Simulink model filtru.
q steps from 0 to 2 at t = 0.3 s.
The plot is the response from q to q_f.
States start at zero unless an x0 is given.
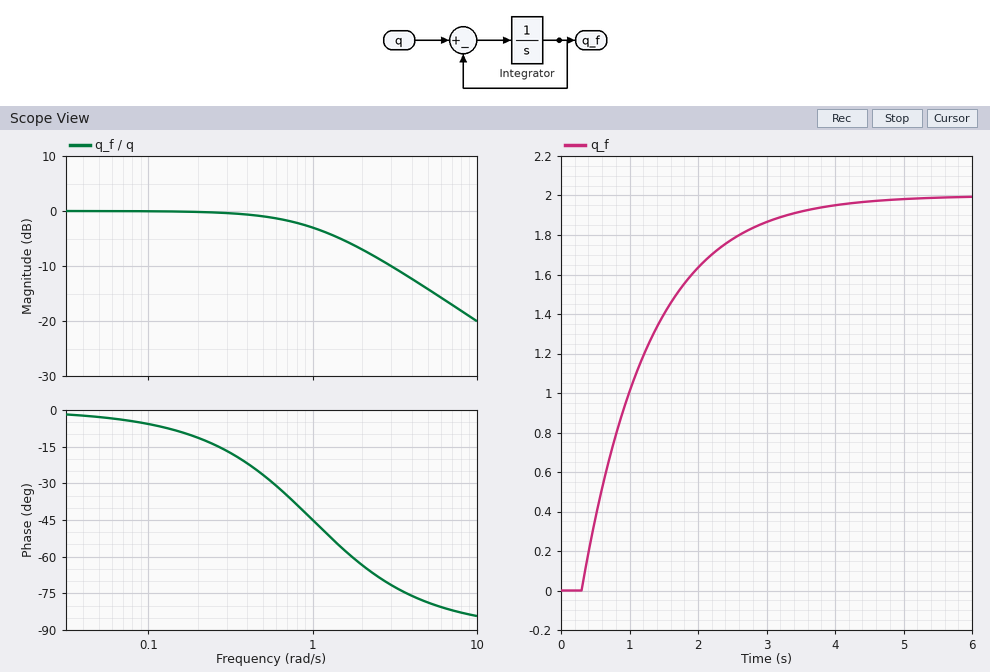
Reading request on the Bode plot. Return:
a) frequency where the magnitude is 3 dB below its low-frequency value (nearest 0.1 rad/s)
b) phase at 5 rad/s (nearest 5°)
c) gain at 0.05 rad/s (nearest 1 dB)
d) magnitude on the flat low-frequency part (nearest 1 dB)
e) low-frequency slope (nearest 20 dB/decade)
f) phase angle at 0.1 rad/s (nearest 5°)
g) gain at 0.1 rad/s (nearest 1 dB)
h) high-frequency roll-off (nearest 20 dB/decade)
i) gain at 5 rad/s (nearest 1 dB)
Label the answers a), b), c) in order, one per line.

a) 1.0 rad/s
b) -80°
c) 0 dB
d) 0 dB
e) 0 dB/decade
f) -5°
g) 0 dB
h) -20 dB/decade
i) -14 dB
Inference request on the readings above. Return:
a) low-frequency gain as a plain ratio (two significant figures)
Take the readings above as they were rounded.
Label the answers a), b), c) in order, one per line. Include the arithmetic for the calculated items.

a) 10^(0 / 20) = 1.0
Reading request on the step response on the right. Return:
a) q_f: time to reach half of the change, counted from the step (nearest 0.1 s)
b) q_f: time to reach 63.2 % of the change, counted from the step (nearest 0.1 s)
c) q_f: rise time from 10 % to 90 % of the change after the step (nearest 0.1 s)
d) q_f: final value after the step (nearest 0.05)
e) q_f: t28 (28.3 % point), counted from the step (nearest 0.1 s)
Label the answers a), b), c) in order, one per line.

a) 0.7 s
b) 1.0 s
c) 2.2 s
d) 2.00
e) 0.3 s
